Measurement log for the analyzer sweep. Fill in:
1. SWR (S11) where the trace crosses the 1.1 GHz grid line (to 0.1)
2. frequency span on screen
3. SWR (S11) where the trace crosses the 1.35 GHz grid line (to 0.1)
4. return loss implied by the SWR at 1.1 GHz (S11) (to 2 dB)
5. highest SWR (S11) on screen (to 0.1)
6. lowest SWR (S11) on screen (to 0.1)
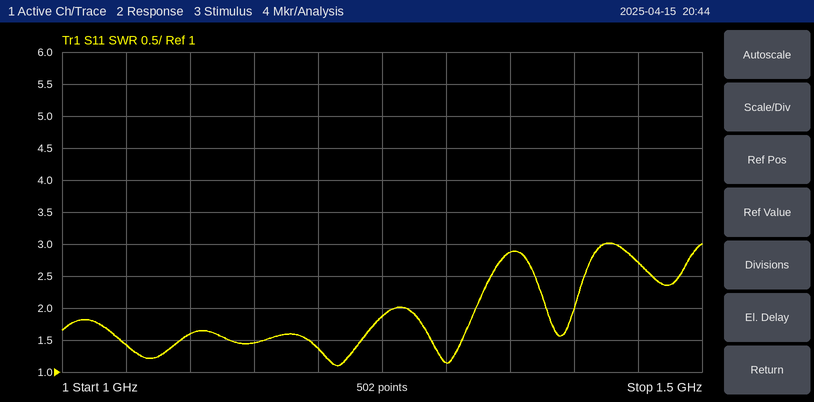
1.6
500 MHz
2.9
12 dB
3.0
1.1
